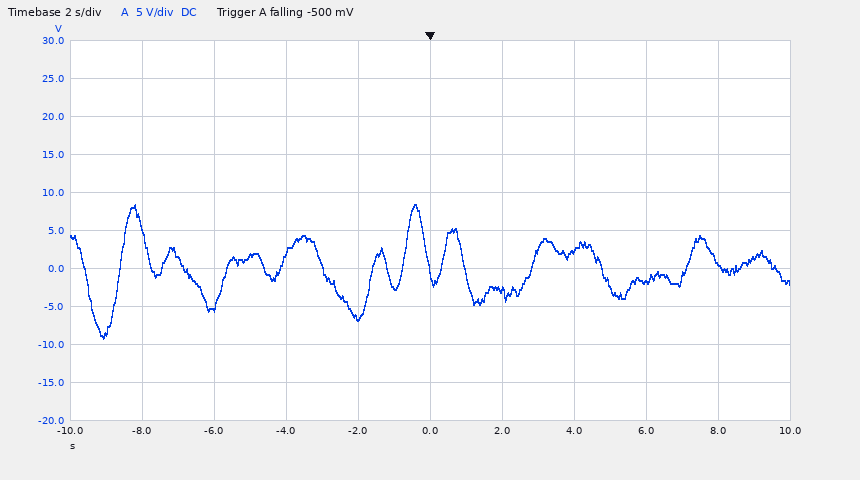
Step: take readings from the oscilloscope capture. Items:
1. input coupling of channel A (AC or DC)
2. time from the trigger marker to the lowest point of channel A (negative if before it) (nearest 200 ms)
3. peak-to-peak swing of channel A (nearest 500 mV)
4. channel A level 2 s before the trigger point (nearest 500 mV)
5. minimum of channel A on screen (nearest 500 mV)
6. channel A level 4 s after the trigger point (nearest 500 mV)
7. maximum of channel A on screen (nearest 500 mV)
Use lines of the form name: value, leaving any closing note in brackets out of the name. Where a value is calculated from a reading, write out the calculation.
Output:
input coupling of channel A: DC
time from the trigger marker to the lowest point of channel A (negative if before it): -9.0 s
peak-to-peak swing of channel A: 8.5 V − (-9.0 V) = 17.5 V
channel A level 2 s before the trigger point: -6.5 V
minimum of channel A on screen: -9.0 V
channel A level 4 s after the trigger point: 2.5 V
maximum of channel A on screen: 8.5 V
